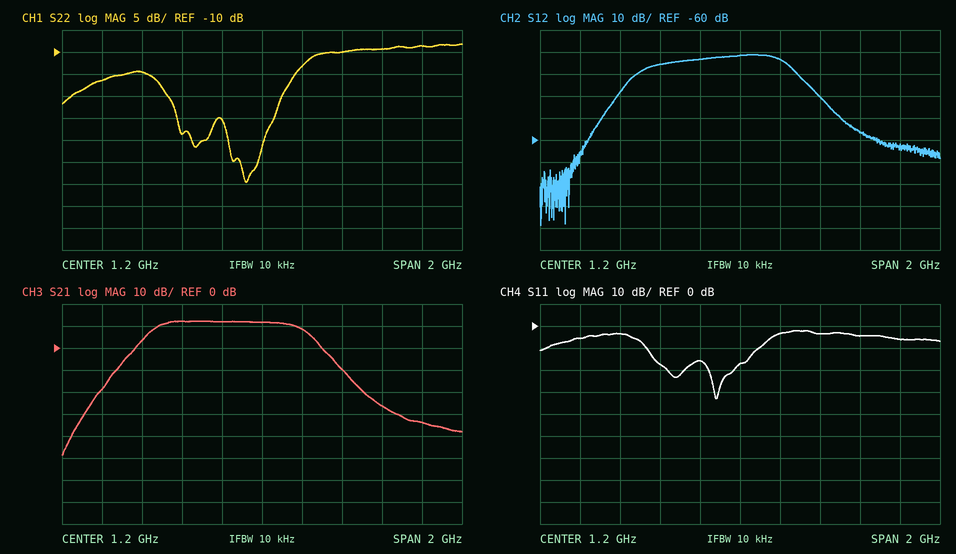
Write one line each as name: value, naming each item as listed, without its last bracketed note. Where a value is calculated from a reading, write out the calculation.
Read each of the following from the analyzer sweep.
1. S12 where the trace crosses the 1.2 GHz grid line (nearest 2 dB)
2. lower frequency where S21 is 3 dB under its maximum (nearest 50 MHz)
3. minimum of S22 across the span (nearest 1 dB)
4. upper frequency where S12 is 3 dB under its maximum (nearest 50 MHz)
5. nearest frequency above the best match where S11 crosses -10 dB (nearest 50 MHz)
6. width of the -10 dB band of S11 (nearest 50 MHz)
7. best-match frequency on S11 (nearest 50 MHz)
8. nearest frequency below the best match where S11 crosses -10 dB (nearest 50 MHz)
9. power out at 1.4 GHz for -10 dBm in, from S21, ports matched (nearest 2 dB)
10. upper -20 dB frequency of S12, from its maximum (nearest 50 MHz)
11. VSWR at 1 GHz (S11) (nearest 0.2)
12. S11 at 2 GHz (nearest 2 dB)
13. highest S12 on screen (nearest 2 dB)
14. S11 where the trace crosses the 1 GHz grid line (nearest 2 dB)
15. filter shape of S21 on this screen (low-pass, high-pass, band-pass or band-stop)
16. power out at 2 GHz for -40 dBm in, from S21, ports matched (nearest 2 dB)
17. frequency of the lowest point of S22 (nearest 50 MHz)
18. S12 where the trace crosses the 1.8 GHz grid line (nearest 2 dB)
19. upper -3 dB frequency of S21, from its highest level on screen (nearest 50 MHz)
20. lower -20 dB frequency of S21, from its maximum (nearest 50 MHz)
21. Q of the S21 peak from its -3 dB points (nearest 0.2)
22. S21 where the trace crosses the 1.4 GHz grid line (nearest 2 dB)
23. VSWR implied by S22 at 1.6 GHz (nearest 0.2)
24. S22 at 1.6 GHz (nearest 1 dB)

S12 where the trace crosses the 1.2 GHz grid line: -22 dB
lower frequency where S21 is 3 dB under its maximum: 650 MHz
minimum of S22 across the span: -40 dB
upper frequency where S12 is 3 dB under its maximum: 1.40 GHz
nearest frequency above the best match where S11 crosses -10 dB: 1.30 GHz
width of the -10 dB band of S11: 1.30 GHz − 750 MHz = 550 MHz
best-match frequency on S11: 1.10 GHz
nearest frequency below the best match where S11 crosses -10 dB: 750 MHz
power out at 1.4 GHz for -10 dBm in, from S21, ports matched: -10 dBm + (8 dB) = -2 dBm
upper -20 dB frequency of S12, from its maximum: 1.60 GHz
VSWR at 1 GHz (S11): |Γ| = 10^(-16/20) = 0.1585; VSWR = (1 + 0.1585)/(1 − 0.1585) ≈ 1.4
S11 at 2 GHz: -6 dB
highest S12 on screen: -22 dB
S11 where the trace crosses the 1 GHz grid line: -16 dB
filter shape of S21 on this screen: band-pass
power out at 2 GHz for -40 dBm in, from S21, ports matched: -40 dBm + (-34 dB) = -74 dBm
frequency of the lowest point of S22: 1.10 GHz
S12 where the trace crosses the 1.8 GHz grid line: -56 dB
upper -3 dB frequency of S21, from its highest level on screen: 1.40 GHz
lower -20 dB frequency of S21, from its maximum: 500 MHz
Q of the S21 peak from its -3 dB points: 1.025 GHz / 750 MHz ≈ 1.4
S21 where the trace crosses the 1.4 GHz grid line: 8 dB
VSWR implied by S22 at 1.6 GHz: |Γ| = 10^(-10/20) = 0.3162; VSWR = (1 + 0.3162)/(1 − 0.3162) ≈ 1.92, so 2.0 to the nearest 0.2
S22 at 1.6 GHz: -10 dB
